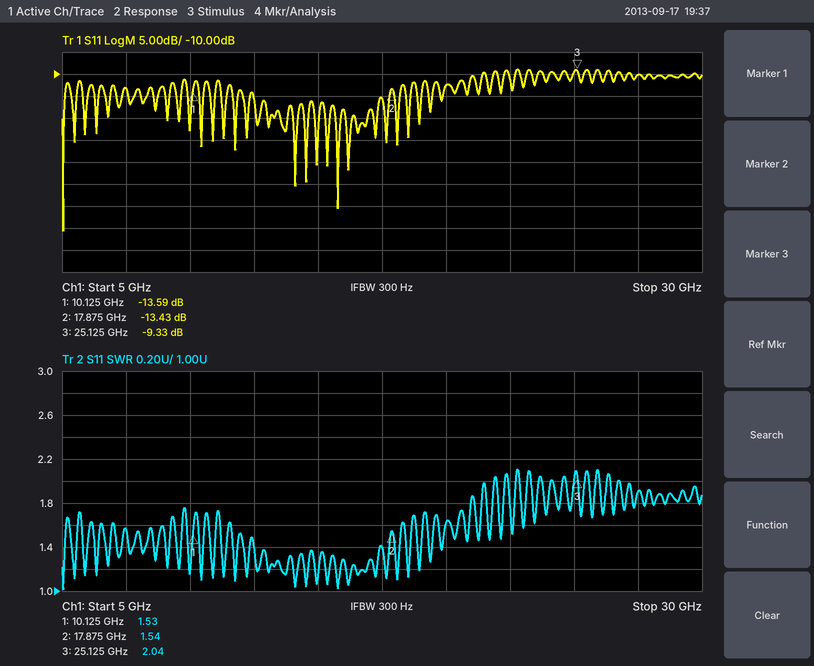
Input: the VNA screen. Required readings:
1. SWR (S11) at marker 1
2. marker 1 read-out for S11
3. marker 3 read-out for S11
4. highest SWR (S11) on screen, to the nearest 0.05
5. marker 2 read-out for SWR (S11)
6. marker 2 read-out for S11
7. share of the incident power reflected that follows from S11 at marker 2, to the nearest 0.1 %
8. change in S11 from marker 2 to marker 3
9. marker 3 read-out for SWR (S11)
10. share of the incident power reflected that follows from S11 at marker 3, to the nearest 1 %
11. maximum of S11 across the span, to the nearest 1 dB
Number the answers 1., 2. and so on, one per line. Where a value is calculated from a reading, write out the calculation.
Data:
1. 1.53
2. -13.59 dB
3. -9.33 dB
4. 2.10
5. 1.54
6. -13.43 dB
7. 10^(-13.43/10) ≈ 4.5 %
8. -9.33 − (-13.43) = 4.10 dB
9. 2.04
10. 10^(-9.33/10) ≈ 12 %
11. -9 dB
